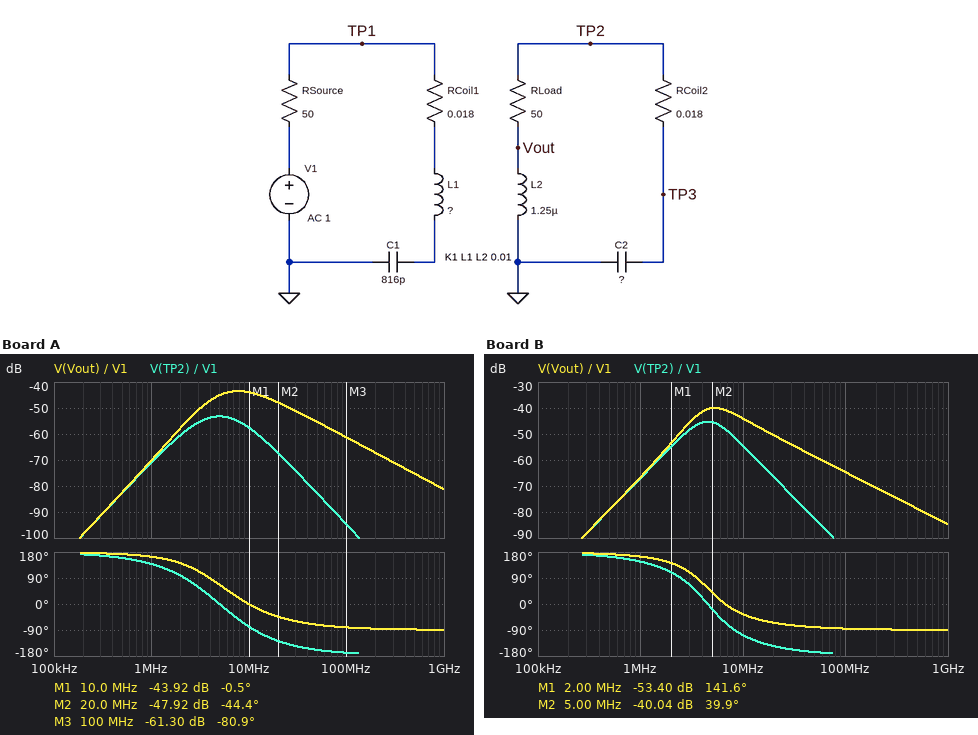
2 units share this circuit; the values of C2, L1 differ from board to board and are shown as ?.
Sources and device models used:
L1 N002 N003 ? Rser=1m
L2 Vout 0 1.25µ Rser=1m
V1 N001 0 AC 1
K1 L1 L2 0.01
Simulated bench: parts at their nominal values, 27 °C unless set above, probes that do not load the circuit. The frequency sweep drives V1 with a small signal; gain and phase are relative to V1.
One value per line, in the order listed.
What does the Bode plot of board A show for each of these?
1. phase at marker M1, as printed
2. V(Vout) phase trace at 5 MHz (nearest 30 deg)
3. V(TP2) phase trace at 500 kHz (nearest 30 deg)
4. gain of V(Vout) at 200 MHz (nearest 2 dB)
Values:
-0.5 deg
60 deg
150 deg
-68 dB
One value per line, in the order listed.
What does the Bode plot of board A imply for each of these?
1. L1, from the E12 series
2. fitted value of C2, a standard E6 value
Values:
680 nH
1.5 nF
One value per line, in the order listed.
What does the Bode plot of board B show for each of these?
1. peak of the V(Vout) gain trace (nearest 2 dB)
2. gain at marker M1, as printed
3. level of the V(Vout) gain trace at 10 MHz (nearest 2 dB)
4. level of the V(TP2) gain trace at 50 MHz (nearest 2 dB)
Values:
-40 dB
-53.40 dB
-44 dB
-82 dB
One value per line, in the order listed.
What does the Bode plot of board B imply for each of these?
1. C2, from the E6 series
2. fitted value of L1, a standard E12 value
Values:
1 nF
1.5 µH
